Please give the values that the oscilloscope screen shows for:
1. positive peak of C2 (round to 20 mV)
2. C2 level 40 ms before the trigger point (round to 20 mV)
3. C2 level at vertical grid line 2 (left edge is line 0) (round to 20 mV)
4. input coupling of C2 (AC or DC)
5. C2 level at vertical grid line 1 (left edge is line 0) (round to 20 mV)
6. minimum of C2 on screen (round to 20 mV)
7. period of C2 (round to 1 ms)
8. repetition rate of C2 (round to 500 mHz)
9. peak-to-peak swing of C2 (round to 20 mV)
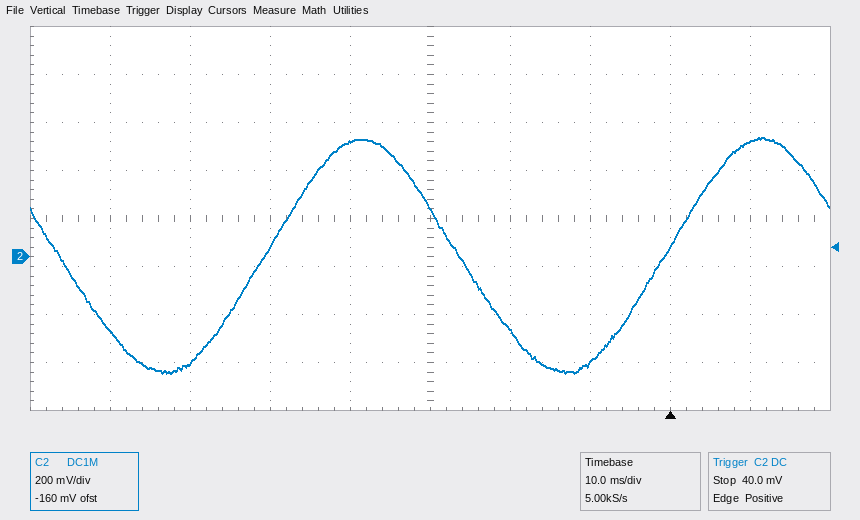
500 mV
480 mV
-440 mV
DC
-300 mV
-480 mV
50 ms
20.0 Hz
980 mV
